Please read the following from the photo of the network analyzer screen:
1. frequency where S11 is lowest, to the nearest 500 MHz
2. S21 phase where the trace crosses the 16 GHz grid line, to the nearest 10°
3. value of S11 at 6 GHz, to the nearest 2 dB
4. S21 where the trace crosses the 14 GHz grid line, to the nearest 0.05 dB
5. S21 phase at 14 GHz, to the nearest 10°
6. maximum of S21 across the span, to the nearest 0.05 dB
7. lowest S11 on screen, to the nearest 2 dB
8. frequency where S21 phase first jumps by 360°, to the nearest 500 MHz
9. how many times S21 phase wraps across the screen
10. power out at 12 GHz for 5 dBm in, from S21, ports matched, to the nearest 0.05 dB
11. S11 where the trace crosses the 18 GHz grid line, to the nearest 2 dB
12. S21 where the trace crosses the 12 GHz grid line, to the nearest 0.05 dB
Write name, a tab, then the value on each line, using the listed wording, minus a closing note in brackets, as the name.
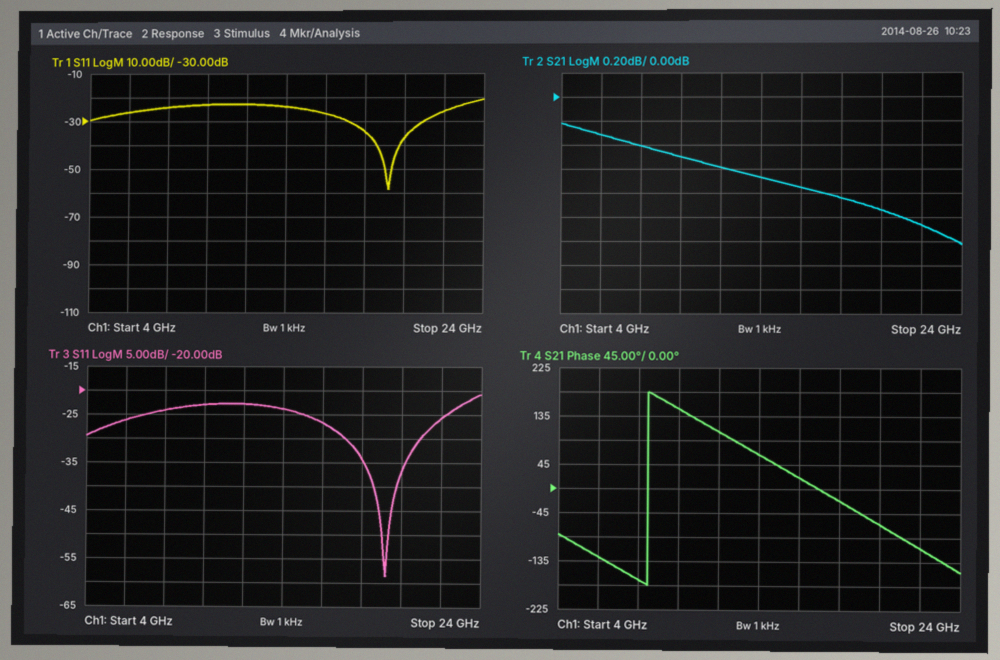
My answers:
frequency where S11 is lowest, to the nearest 500 MHz	19.0 GHz
S21 phase where the trace crosses the 16 GHz grid line, to the nearest 10°	20°
value of S11 at 6 GHz, to the nearest 2 dB	-26 dB
S21 where the trace crosses the 14 GHz grid line, to the nearest 0.05 dB	-0.65 dB
S21 phase at 14 GHz, to the nearest 10°	60°
maximum of S21 across the span, to the nearest 0.05 dB	-0.20 dB
lowest S11 on screen, to the nearest 2 dB	-58 dB
frequency where S21 phase first jumps by 360°, to the nearest 500 MHz	8.5 GHz
how many times S21 phase wraps across the screen	1
power out at 12 GHz for 5 dBm in, from S21, ports matched, to the nearest 0.05 dB	4.40 dBm
S11 where the trace crosses the 18 GHz grid line, to the nearest 2 dB	-34 dB
S21 where the trace crosses the 12 GHz grid line, to the nearest 0.05 dB	-0.60 dB
